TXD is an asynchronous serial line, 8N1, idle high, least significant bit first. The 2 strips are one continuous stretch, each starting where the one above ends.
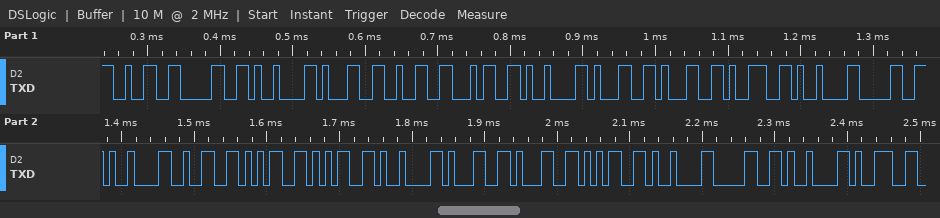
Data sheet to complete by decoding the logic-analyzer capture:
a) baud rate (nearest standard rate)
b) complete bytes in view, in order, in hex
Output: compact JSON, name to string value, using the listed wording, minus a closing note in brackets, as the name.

{"baud rate": "115200 baud", "complete bytes in view, in order, in hex": "32 30 09 31 32 34 09 31 31 39 09 30 09 32 35 35 09 31 31 35 09 30 09 39"}
